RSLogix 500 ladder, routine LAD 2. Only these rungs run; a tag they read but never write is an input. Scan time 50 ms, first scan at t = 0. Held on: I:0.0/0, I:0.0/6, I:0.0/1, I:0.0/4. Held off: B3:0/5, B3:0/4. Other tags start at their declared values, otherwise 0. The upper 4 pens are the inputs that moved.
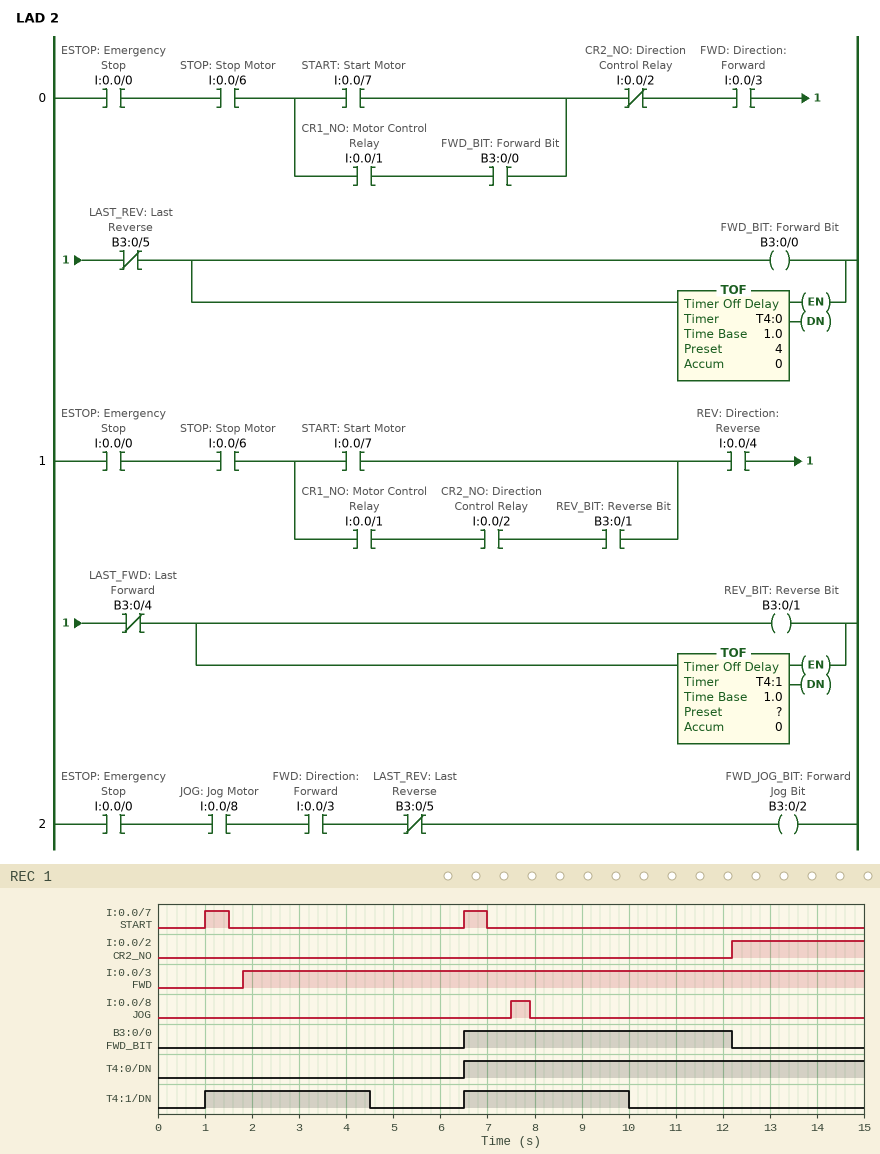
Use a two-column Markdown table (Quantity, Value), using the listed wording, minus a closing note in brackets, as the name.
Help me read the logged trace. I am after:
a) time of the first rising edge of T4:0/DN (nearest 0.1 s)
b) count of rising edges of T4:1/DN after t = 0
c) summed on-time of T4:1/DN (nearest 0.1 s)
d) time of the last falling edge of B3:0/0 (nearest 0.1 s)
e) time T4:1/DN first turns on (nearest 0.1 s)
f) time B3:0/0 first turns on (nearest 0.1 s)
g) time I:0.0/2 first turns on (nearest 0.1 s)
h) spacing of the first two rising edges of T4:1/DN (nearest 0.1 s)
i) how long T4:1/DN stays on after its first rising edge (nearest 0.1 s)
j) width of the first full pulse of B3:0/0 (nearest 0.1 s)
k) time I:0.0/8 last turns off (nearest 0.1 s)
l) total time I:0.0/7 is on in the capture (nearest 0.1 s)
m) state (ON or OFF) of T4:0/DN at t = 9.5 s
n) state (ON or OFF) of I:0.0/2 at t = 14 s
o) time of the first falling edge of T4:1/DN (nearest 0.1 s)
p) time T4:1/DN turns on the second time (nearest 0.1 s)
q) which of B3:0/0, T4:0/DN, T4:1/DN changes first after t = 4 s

| Quantity | Value |
|---|---|
| time of the first rising edge of T4:0/DN | 6.5 s |
| count of rising edges of T4:1/DN after t = 0 | 2 |
| summed on-time of T4:1/DN | 7.0 s |
| time of the last falling edge of B3:0/0 | 12.2 s |
| time T4:1/DN first turns on | 1.0 s |
| time B3:0/0 first turns on | 6.5 s |
| time I:0.0/2 first turns on | 12.2 s |
| spacing of the first two rising edges of T4:1/DN | 5.5 s |
| how long T4:1/DN stays on after its first rising edge | 3.5 s |
| width of the first full pulse of B3:0/0 | 5.7 s |
| time I:0.0/8 last turns off | 7.9 s |
| total time I:0.0/7 is on in the capture | 1.0 s |
| state (ON or OFF) of T4:0/DN at t = 9.5 s | ON |
| state (ON or OFF) of I:0.0/2 at t = 14 s | ON |
| time of the first falling edge of T4:1/DN | 4.5 s |
| time T4:1/DN turns on the second time | 6.5 s |
| which of B3:0/0, T4:0/DN, T4:1/DN changes first after t = 4 s | T4:1/DN |
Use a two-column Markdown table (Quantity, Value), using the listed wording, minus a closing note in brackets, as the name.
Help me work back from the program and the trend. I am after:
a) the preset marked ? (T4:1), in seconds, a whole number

| Quantity | Value |
|---|---|
| the preset marked ? (T4:1), in seconds, a whole number | 3 s |
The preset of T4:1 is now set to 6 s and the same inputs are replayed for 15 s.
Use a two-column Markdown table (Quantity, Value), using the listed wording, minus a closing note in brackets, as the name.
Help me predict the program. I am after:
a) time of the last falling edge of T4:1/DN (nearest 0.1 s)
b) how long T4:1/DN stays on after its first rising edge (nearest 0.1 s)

| Quantity | Value |
|---|---|
| time of the last falling edge of T4:1/DN | 13.0 s |
| how long T4:1/DN stays on after its first rising edge | 12.0 s |
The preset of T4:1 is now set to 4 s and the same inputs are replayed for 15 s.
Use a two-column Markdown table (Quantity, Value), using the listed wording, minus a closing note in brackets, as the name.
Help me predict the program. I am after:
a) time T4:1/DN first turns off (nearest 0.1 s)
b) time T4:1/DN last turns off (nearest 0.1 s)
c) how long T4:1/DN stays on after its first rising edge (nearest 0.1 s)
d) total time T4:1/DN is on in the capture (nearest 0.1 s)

| Quantity | Value |
|---|---|
| time T4:1/DN first turns off | 5.5 s |
| time T4:1/DN last turns off | 11.0 s |
| how long T4:1/DN stays on after its first rising edge | 4.5 s |
| total time T4:1/DN is on in the capture | 9.0 s |
